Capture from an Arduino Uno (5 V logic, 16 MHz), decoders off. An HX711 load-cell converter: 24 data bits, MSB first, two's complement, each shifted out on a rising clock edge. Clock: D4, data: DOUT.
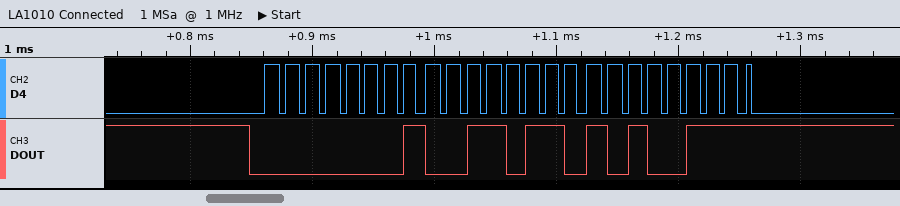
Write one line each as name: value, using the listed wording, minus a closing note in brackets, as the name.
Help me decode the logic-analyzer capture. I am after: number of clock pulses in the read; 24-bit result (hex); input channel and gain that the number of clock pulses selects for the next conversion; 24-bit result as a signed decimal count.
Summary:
number of clock pulses in the read: 25
24-bit result: 0x0136A7
input channel and gain that the number of clock pulses selects for the next conversion: channel A, gain 128
24-bit result as a signed decimal count: 79527
